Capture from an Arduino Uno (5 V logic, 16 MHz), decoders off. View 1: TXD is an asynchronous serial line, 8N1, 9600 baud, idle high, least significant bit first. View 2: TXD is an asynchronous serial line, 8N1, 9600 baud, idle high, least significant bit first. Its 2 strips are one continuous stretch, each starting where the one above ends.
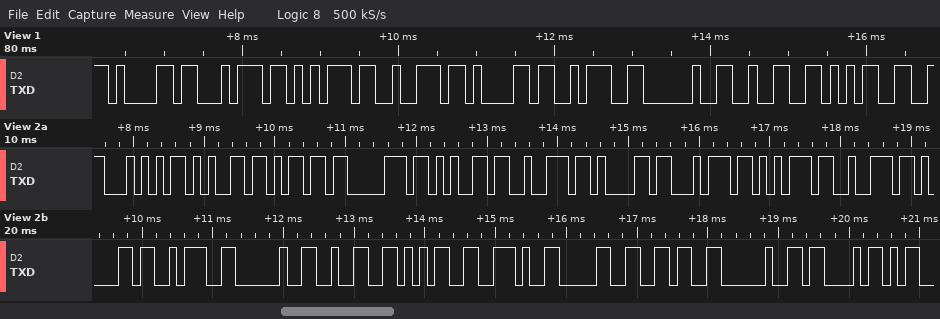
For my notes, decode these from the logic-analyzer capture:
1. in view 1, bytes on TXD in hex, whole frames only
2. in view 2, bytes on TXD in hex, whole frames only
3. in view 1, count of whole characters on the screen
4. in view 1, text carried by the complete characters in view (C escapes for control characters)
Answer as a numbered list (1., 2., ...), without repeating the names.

1. 61 74 75 72 61 3A 20 32 35
2. 54 65 6D 70 65 72 61 74 75 72 61 3A 20 32 35 2E 30 36 20 43
3. 9
4. "atura: 25"
